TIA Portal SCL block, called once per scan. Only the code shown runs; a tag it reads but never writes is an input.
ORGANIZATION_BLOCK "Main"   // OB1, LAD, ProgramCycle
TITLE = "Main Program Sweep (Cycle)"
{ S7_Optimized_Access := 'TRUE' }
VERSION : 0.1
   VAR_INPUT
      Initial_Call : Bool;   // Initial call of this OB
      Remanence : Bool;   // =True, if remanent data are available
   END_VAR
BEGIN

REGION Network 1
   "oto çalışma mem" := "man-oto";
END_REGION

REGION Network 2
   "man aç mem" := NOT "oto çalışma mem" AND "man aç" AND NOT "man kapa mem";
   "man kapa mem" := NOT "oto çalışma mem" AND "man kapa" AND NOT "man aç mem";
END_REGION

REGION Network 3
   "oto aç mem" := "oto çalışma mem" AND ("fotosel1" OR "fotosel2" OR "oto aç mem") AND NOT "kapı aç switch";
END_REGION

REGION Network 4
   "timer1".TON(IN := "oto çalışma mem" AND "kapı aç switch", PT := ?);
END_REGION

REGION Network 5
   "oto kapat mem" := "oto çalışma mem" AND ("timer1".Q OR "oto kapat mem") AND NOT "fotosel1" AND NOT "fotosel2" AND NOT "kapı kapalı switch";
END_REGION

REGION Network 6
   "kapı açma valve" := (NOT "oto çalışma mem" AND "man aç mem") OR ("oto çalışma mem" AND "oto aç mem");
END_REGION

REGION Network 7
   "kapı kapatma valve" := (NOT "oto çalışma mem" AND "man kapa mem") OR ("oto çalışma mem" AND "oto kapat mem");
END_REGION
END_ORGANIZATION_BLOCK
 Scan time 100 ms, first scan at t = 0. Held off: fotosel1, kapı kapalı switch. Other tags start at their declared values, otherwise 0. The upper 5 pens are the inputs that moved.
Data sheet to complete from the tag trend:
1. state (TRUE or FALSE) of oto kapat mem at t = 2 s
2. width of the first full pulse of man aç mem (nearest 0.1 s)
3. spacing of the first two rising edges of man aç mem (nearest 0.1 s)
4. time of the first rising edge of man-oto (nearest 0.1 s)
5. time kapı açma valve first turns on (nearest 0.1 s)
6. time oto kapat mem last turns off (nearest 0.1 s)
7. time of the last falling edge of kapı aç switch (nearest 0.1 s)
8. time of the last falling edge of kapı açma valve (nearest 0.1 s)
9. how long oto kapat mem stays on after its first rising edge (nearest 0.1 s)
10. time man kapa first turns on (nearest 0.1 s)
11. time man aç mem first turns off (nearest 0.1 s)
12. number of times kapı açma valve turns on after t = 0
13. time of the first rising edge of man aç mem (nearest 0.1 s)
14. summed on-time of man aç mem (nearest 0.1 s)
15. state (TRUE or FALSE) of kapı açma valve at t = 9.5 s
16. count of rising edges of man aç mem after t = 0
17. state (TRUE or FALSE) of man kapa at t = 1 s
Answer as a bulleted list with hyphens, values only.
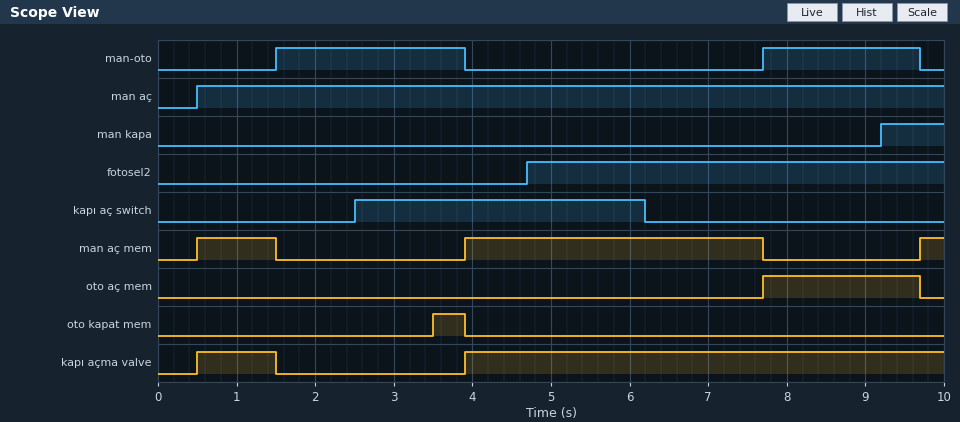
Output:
- FALSE
- 1.0 s
- 3.4 s
- 1.5 s
- 0.5 s
- 3.9 s
- 6.2 s
- 1.5 s
- 0.4 s
- 9.2 s
- 1.5 s
- 2
- 0.5 s
- 5.1 s
- TRUE
- 3
- FALSE
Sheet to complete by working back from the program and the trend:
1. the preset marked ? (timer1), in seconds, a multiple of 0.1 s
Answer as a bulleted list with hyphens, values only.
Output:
- 1.0 s
